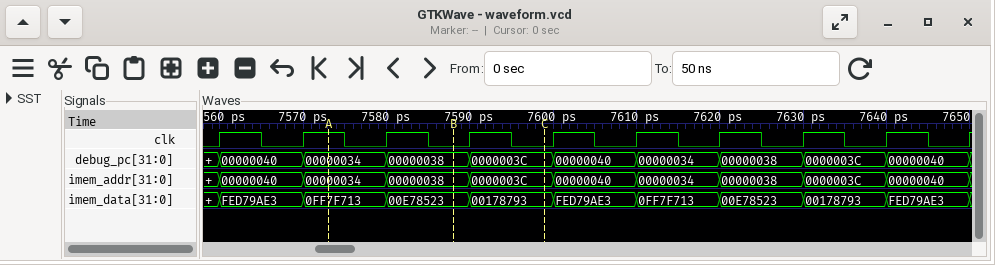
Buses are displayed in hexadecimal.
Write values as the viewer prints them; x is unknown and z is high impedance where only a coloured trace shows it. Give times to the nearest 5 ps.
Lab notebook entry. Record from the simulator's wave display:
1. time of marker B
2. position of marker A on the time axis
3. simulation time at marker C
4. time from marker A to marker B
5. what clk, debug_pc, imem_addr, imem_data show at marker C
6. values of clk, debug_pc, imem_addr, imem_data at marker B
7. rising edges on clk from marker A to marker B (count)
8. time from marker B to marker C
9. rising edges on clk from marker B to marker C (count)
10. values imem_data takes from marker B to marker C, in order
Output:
7590 ps
7575 ps
7600 ps
15 ps
clk=0, debug_pc=0000003C, imem_addr=0000003C, imem_data=00178793
clk=0, debug_pc=00000038, imem_addr=00000038, imem_data=00E78523
1
10 ps
1
00E78523, 00178793
